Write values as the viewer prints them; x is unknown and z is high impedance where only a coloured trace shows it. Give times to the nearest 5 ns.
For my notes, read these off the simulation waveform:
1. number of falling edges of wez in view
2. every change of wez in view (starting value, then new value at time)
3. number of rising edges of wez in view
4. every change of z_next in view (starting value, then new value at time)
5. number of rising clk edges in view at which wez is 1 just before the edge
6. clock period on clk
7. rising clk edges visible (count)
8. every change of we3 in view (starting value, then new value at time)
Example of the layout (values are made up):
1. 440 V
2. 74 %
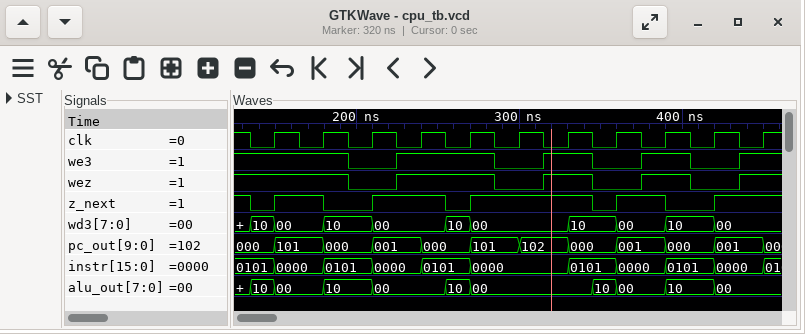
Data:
1. 4
2. 1, 0 at 195 ns, 1 at 225 ns, 0 at 285 ns, 1 at 315 ns, 0 at 345 ns, 1 at 375 ns, 0 at 405 ns, 1 at 435 ns
3. 4
4. 1, 0 at 135 ns, 1 at 150 ns, 0 at 180 ns, 1 at 210 ns, 0 at 255 ns, 1 at 270 ns, 0 at 345 ns, 1 at 360 ns, 0 at 390 ns, 1 at 420 ns
5. 7
6. 30 ns
7. 11
8. 1, 0 at 195 ns, 1 at 225 ns, 0 at 285 ns, 1 at 315 ns, 0 at 345 ns, 1 at 375 ns, 0 at 405 ns, 1 at 435 ns
